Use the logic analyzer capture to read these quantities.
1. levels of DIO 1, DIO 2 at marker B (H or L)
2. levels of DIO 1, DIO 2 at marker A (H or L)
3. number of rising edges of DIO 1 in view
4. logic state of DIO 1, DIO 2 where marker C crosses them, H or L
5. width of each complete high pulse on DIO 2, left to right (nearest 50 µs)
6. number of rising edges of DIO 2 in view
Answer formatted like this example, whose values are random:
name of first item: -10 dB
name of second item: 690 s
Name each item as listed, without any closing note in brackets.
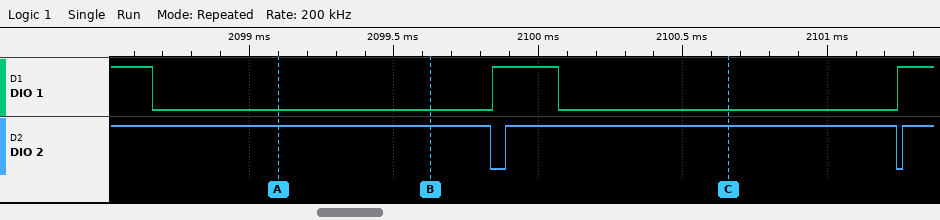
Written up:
levels of DIO 1, DIO 2 at marker B: DIO 1=L, DIO 2=H
levels of DIO 1, DIO 2 at marker A: DIO 1=L, DIO 2=H
number of rising edges of DIO 1 in view: 2
logic state of DIO 1, DIO 2 where marker C crosses them, H or L: DIO 1=L, DIO 2=H
width of each complete high pulse on DIO 2, left to right: 1350 µs
number of rising edges of DIO 2 in view: 2
